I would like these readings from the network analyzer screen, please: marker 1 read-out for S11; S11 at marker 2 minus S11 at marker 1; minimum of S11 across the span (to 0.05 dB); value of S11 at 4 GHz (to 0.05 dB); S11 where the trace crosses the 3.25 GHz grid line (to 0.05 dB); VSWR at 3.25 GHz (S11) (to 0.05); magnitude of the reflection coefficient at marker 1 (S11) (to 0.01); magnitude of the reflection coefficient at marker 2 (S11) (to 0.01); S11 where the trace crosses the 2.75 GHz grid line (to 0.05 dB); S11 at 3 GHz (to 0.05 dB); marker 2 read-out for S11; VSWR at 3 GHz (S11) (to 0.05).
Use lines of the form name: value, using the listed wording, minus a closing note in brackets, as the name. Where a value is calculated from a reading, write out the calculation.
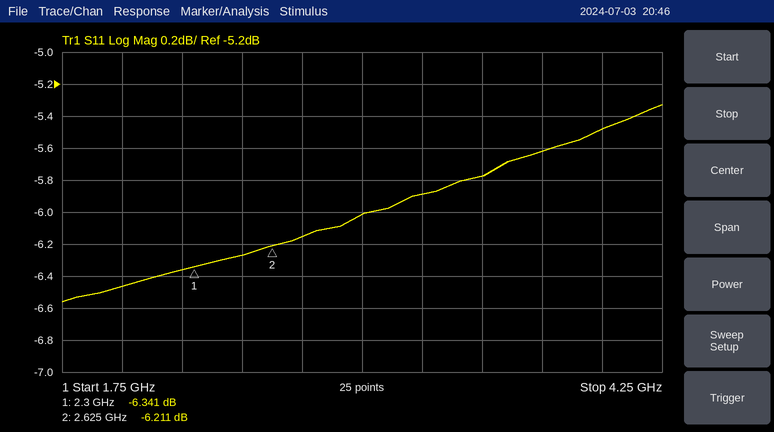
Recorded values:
marker 1 read-out for S11: -6.341 dB
S11 at marker 2 minus S11 at marker 1: -6.211 − (-6.341) = 0.130 dB
minimum of S11 across the span: -6.55 dB
value of S11 at 4 GHz: -5.50 dB
S11 where the trace crosses the 3.25 GHz grid line: -5.90 dB
VSWR at 3.25 GHz (S11): |Γ| = 10^(-5.9/20) = 0.5070; VSWR = (1 + 0.5070)/(1 − 0.5070) ≈ 3.06, so 3.05 to the nearest 0.05
magnitude of the reflection coefficient at marker 1 (S11): 10^(-6.341/20) ≈ 0.48
magnitude of the reflection coefficient at marker 2 (S11): 10^(-6.211/20) ≈ 0.49
S11 where the trace crosses the 2.75 GHz grid line: -6.15 dB
S11 at 3 GHz: -6.00 dB
marker 2 read-out for S11: -6.211 dB
VSWR at 3 GHz (S11): |Γ| = 10^(-6/20) = 0.5012; VSWR = (1 + 0.5012)/(1 − 0.5012) ≈ 3.01, so 3.00 to the nearest 0.05
